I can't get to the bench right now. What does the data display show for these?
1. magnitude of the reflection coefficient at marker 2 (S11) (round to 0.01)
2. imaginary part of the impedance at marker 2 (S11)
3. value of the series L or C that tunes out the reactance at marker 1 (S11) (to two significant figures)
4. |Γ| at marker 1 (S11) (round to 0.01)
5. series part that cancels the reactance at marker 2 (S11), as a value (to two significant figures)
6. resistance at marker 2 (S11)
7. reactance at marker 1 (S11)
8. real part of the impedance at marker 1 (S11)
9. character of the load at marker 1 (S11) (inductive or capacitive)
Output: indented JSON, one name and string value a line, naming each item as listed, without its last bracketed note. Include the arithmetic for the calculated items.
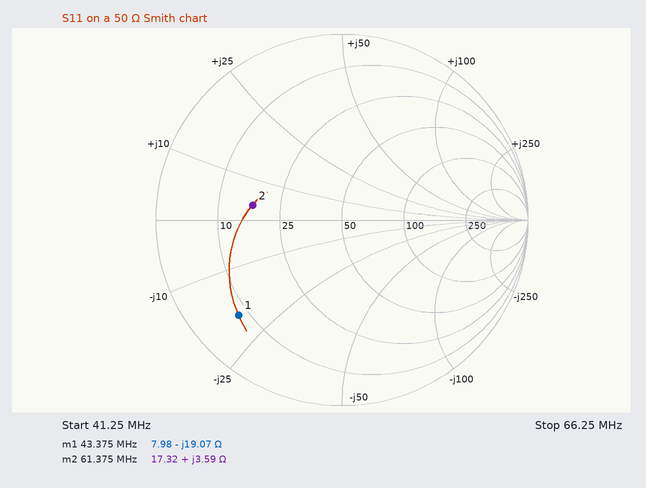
{
  "magnitude of the reflection coefficient at marker 2 (S11)": "0.49",
  "imaginary part of the impedance at marker 2": "+3.59 Ω",
  "value of the series L or C that tunes out the reactance at marker 1 (S11)": "L = 19.07 Ω/(2π × 43.375 MHz) ≈ 70 nH",
  "|Γ| at marker 1 (S11)": "0.76",
  "series part that cancels the reactance at marker 2 (S11), as a value": "C = 1/(2π × 61.375 MHz × 3.59 Ω) ≈ 722 pF, so 720 pF to two significant figures",
  "resistance at marker 2": "17.32 Ω",
  "reactance at marker 1": "-19.07 Ω",
  "real part of the impedance at marker 1": "7.98 Ω",
  "character of the load at marker 1 (S11)": "capacitive"
}
